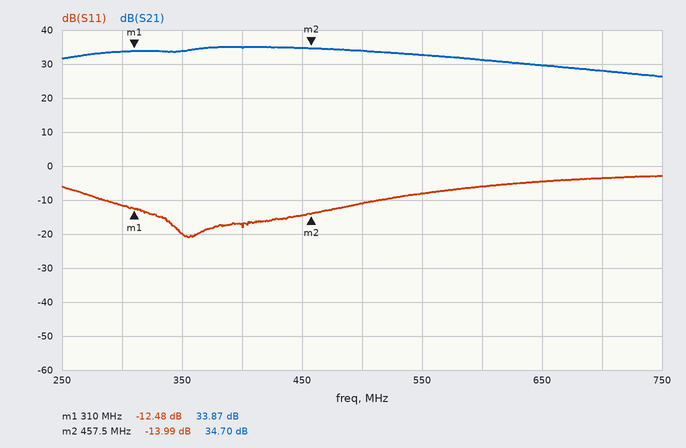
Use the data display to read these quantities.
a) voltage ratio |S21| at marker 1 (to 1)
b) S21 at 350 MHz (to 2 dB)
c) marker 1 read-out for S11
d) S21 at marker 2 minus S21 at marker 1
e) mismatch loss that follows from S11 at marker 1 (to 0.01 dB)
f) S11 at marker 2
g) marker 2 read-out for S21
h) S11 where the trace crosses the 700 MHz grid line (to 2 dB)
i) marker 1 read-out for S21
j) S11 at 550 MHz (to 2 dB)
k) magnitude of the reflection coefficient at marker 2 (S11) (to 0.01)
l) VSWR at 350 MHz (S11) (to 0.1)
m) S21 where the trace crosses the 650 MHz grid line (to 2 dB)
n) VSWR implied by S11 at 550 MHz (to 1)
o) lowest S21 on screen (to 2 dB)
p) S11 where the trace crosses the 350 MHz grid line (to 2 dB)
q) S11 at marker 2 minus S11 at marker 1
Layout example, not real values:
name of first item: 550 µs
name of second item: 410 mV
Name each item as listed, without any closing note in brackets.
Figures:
voltage ratio |S21| at marker 1: 49
S21 at 350 MHz: 34 dB
marker 1 read-out for S11: -12.48 dB
S21 at marker 2 minus S21 at marker 1: 0.83 dB
mismatch loss that follows from S11 at marker 1: 0.25 dB
S11 at marker 2: -13.99 dB
marker 2 read-out for S21: 34.70 dB
S11 where the trace crosses the 700 MHz grid line: -4 dB
marker 1 read-out for S21: 33.87 dB
S11 at 550 MHz: -8 dB
magnitude of the reflection coefficient at marker 2 (S11): 0.20
VSWR at 350 MHz (S11): 1.2
S21 where the trace crosses the 650 MHz grid line: 30 dB
VSWR implied by S11 at 550 MHz: 2
lowest S21 on screen: 26 dB
S11 where the trace crosses the 350 MHz grid line: -20 dB
S11 at marker 2 minus S11 at marker 1: -1.51 dB
